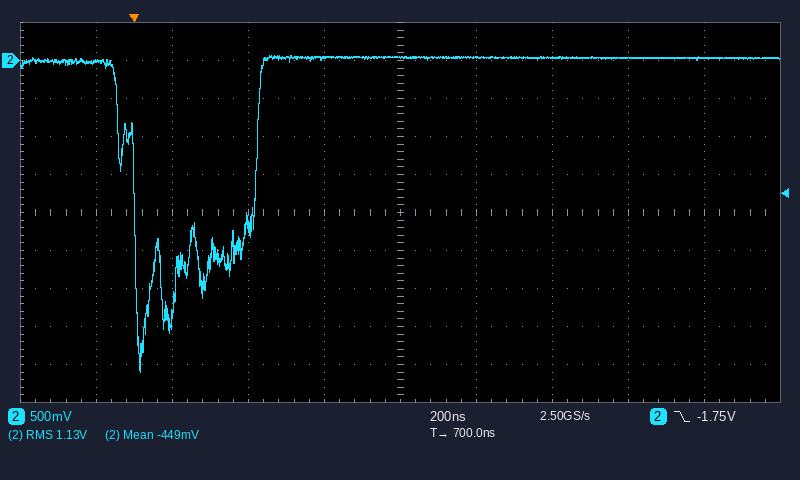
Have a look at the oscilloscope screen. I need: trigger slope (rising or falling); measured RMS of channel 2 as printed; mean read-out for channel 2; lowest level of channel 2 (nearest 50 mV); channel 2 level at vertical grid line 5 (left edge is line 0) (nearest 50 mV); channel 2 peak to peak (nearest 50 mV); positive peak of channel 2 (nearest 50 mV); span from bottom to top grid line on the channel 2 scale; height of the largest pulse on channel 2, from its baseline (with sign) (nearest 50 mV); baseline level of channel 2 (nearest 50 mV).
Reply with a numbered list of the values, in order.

1. falling
2. 1.13 V
3. -449 mV
4. -4.10 V
5. 50 mV
6. 4.15 V
7. 50 mV
8. 5 V
9. -4.15 V
10. 50 mV
